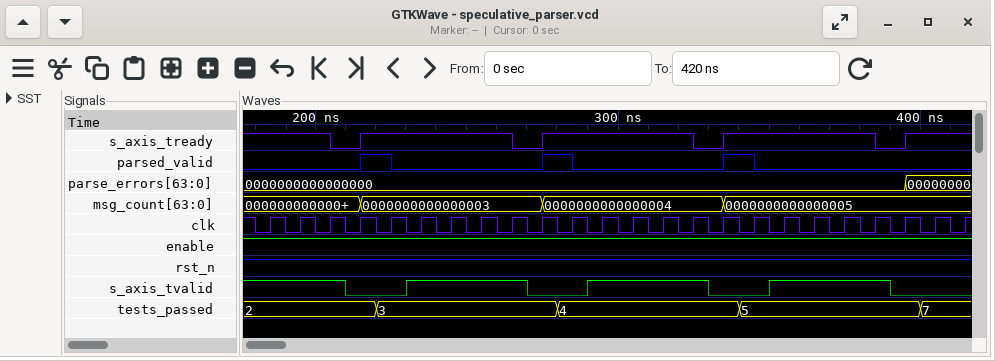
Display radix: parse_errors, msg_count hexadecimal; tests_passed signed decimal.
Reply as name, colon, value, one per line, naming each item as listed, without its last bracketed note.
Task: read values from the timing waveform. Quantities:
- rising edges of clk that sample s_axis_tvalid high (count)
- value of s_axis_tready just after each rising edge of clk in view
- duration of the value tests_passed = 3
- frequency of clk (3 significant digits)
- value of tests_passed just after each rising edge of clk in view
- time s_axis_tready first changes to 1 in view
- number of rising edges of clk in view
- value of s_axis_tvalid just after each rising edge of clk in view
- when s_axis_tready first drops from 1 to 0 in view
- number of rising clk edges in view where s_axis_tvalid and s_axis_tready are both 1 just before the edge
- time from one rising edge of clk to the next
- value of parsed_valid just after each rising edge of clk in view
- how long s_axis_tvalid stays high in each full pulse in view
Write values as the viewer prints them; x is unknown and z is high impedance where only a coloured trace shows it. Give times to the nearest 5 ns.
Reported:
rising edges of clk that sample s_axis_tvalid high: 15
value of s_axis_tready just after each rising edge of clk in view: 1 1 0 1 1 1 1 1 0 1 1 1 1 1 0 1 1 1 1 1 0 1 1 1
duration of the value tests_passed = 3: 60 ns
frequency of clk: 100 MHz
value of tests_passed just after each rising edge of clk in view: 2, 2, 2, 2, 3, 3, 3, 3, 3, 3, 4, 4, 4, 4, 4, 4, 5, 5, 5, 5, 5, 5, 7, 7
time s_axis_tready first changes to 1 in view: 215 ns
number of rising edges of clk in view: 24
value of s_axis_tvalid just after each rising edge of clk in view: 1 1 1 0 0 1 1 1 1 0 0 1 1 1 1 0 0 1 1 1 1 0 0 0
when s_axis_tready first drops from 1 to 0 in view: 205 ns
number of rising clk edges in view where s_axis_tvalid and s_axis_tready are both 1 just before the edge: 15
time from one rising edge of clk to the next: 10 ns
value of parsed_valid just after each rising edge of clk in view: 0 0 0 1 0 0 0 0 0 1 0 0 0 0 0 1 0 0 0 0 0 0 0 0
how long s_axis_tvalid stays high in each full pulse in view: 40 ns, 40 ns, 40 ns
